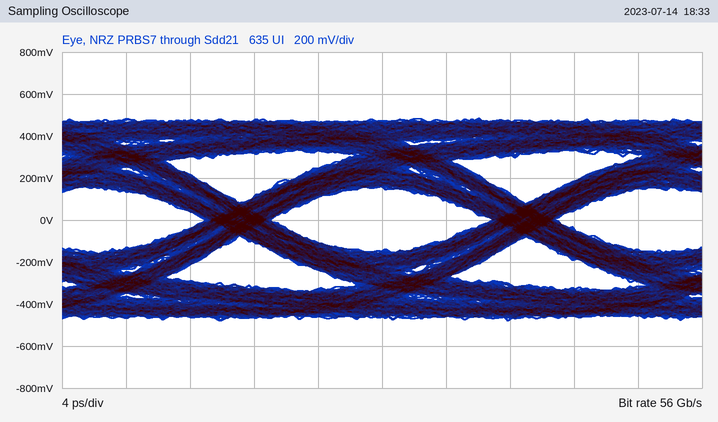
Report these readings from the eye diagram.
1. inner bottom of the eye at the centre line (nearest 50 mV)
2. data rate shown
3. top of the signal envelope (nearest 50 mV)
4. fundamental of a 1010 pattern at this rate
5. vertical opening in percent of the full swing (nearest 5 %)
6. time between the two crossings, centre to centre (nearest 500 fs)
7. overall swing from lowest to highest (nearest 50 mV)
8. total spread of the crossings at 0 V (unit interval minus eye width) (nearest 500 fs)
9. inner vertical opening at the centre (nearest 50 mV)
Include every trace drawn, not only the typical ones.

-150 mV
56 Gb/s
500 mV
28 GHz
30 %
18.0 ps
950 mV
4.0 ps
300 mV
